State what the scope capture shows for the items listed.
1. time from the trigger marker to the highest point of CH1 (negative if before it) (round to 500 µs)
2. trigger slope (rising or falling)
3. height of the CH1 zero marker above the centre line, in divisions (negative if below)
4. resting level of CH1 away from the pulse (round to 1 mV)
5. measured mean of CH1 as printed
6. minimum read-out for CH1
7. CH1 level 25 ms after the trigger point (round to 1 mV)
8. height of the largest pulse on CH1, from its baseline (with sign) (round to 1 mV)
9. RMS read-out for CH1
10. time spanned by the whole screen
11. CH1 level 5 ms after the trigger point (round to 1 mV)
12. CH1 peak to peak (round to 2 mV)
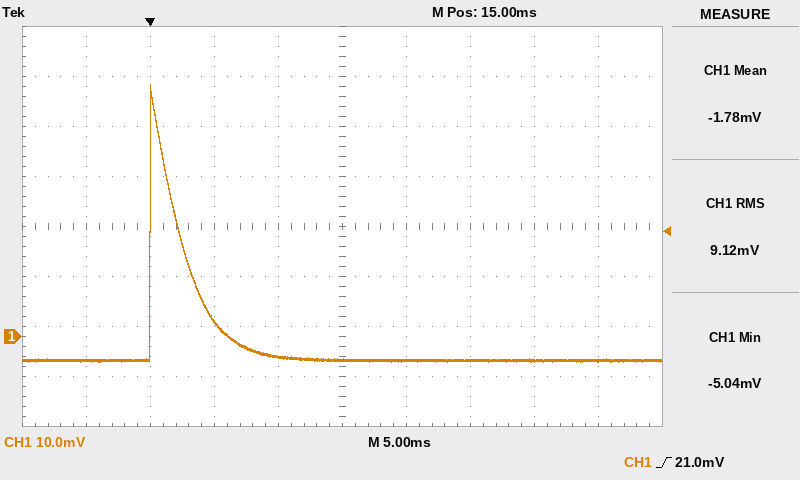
0.0 ms
rising
-2.2 div
-5 mV
-1.78 mV
-5.04 mV
-5 mV
+55 mV
9.12 mV
50 ms
3 mV
56 mV
